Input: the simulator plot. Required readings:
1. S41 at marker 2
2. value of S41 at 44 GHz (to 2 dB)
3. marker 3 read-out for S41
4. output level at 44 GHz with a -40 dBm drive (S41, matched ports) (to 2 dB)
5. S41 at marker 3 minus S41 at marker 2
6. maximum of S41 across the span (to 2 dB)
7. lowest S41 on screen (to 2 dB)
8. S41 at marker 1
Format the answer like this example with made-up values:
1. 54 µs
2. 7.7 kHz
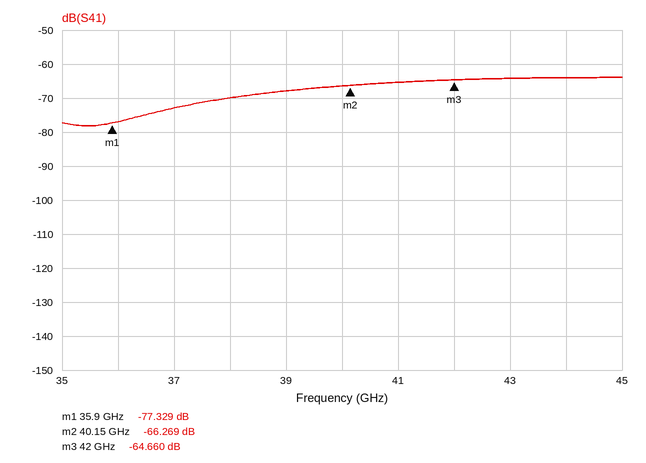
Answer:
1. -66.269 dB
2. -64 dB
3. -64.660 dB
4. -104 dBm
5. 1.609 dB
6. -64 dB
7. -78 dB
8. -77.329 dB
